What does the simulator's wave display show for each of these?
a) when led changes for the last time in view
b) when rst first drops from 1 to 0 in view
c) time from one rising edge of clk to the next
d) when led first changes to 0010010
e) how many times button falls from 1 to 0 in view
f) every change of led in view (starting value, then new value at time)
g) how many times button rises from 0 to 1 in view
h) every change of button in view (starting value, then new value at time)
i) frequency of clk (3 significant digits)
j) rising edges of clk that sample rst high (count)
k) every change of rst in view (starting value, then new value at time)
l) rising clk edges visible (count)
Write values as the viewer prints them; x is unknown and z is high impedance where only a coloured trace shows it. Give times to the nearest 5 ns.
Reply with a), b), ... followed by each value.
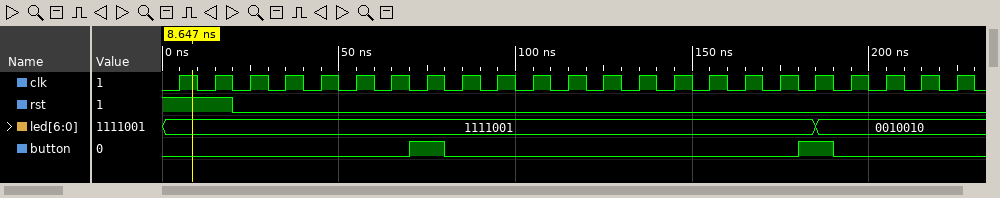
a) 185 ns
b) 20 ns
c) 10 ns
d) 185 ns
e) 2
f) 1111001, 0010010 at 185 ns
g) 2
h) 0, 1 at 70 ns, 0 at 80 ns, 1 at 180 ns, 0 at 190 ns
i) 100 MHz
j) 2
k) 1, 0 at 20 ns
l) 23
